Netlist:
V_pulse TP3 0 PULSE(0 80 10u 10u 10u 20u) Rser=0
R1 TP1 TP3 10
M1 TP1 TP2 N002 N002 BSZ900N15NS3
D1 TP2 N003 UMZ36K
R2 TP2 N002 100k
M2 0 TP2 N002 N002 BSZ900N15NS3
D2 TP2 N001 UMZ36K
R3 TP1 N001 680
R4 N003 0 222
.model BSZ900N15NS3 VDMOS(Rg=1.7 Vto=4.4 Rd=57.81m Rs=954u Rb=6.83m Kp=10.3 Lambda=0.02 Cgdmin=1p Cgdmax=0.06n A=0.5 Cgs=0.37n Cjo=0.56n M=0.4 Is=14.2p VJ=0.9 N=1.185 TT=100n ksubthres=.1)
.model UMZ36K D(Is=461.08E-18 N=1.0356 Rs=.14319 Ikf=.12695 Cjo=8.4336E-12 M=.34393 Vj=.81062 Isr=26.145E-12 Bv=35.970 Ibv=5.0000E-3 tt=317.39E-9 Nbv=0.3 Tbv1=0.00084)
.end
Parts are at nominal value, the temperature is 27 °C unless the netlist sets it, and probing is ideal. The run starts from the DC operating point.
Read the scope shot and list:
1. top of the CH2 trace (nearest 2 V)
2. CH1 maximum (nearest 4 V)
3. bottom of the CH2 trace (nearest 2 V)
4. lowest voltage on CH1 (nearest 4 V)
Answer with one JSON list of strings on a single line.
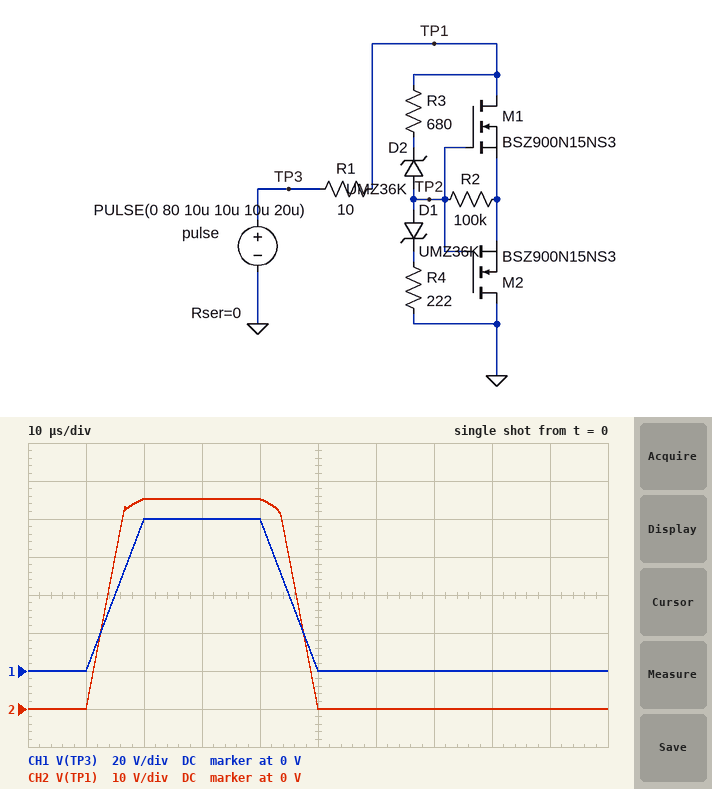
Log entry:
["56 V", "80 V", "0 V", "0 V"]
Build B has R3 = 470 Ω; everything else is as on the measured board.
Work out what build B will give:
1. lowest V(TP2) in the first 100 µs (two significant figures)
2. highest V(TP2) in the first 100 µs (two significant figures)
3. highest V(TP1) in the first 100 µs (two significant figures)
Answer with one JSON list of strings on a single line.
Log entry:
["-15 V", "5.5 V", "51 V"]
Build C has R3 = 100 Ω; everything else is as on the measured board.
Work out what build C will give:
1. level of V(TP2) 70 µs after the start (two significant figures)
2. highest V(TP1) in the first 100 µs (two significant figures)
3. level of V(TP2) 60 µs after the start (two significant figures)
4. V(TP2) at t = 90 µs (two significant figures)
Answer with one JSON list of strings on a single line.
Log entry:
["-14 V", "44 V", "-13 V", "-14 V"]
